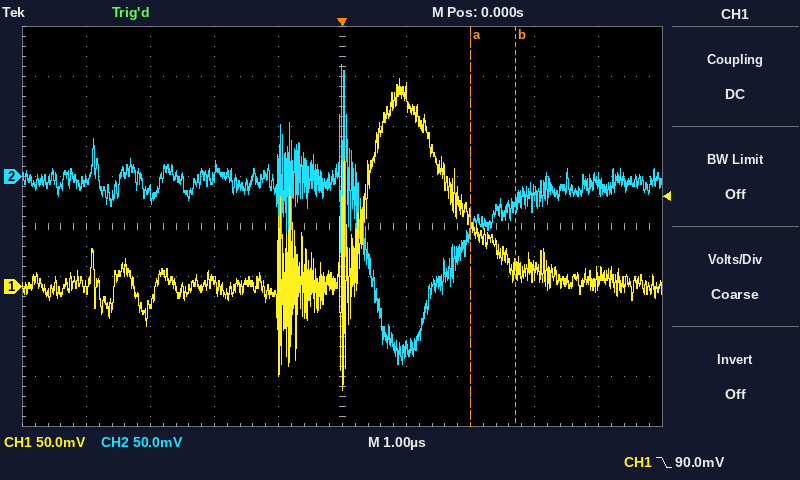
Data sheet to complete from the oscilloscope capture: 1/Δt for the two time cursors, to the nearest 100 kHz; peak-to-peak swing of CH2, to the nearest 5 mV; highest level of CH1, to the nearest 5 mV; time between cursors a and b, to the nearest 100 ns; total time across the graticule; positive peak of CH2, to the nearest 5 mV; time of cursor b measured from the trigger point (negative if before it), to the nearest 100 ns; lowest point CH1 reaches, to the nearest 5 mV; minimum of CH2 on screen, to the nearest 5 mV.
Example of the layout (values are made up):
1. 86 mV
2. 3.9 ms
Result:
1. 1.4 MHz
2. 300 mV
3. 210 mV
4. 700 ns
5. 10 µs
6. 110 mV
7. +2.7 µs
8. -105 mV
9. -190 mV
